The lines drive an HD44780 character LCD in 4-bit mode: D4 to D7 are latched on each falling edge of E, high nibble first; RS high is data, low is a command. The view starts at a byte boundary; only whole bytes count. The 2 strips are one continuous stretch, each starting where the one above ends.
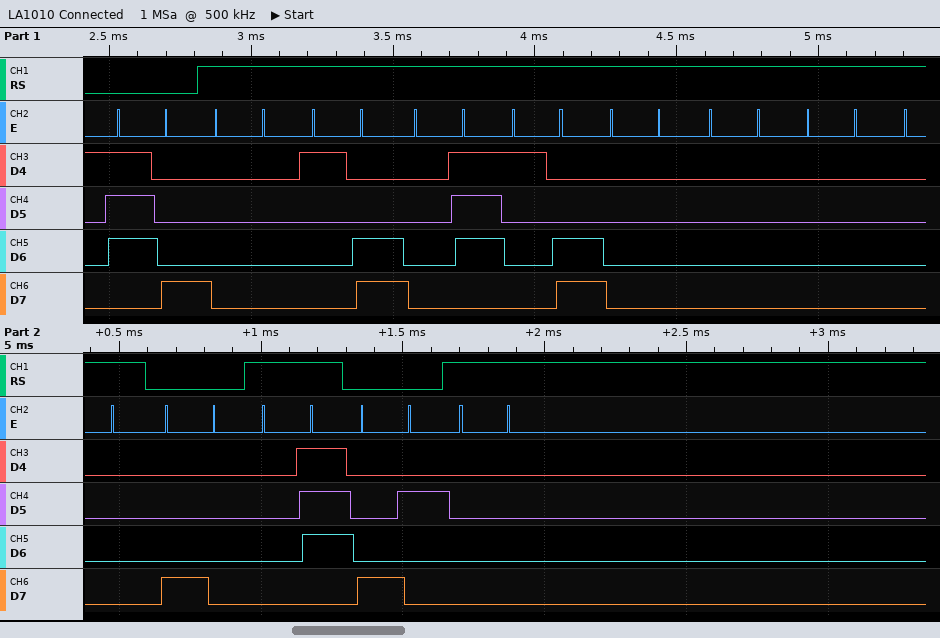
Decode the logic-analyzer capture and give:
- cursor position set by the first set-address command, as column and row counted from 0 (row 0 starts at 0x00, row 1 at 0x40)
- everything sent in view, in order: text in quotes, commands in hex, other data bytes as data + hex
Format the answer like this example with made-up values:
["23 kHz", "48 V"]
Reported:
["column 0, row 0", "0x78 data 00 1C 07 1C 00 00 00 00 0x80 data 07 0x82 data 00"]
